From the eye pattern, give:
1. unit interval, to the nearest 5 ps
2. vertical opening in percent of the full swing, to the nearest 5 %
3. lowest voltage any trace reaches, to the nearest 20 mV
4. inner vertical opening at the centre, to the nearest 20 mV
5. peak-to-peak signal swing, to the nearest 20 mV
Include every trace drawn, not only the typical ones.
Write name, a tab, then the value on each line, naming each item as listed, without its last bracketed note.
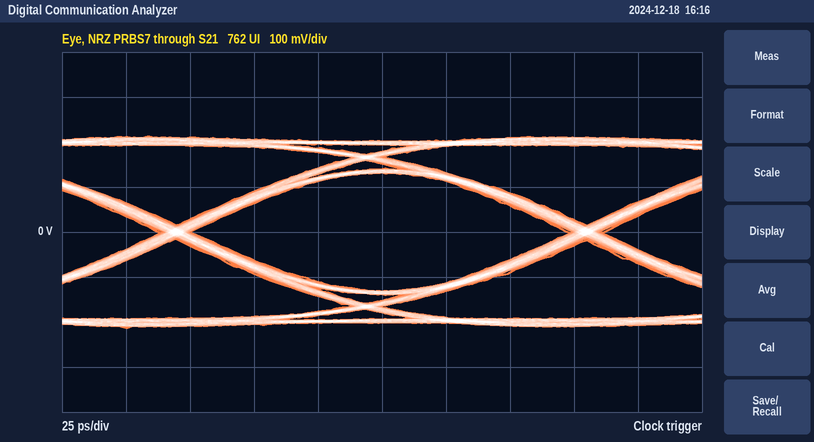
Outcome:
unit interval, to the nearest 5 ps	160 ps
vertical opening in percent of the full swing, to the nearest 5 %	60 %
lowest voltage any trace reaches, to the nearest 20 mV	-220 mV
inner vertical opening at the centre, to the nearest 20 mV	260 mV
peak-to-peak signal swing, to the nearest 20 mV	420 mV
